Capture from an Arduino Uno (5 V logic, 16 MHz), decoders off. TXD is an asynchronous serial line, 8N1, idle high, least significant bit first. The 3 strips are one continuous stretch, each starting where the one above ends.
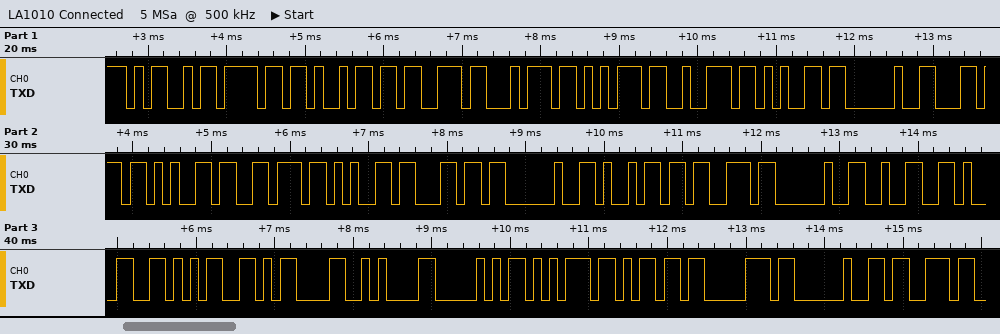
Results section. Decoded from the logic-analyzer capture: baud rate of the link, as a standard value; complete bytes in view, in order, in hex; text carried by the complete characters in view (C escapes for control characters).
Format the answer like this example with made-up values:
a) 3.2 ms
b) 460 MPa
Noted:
a) 9600 baud
b) 4D 6F 69 73 74 75 72 65 20 6C 65 76 65 6C 20 69 73 20 32 31 35 0D 0A 50 75 6D 70 20 73
c) "Moisture level is 215\r\nPump s"
